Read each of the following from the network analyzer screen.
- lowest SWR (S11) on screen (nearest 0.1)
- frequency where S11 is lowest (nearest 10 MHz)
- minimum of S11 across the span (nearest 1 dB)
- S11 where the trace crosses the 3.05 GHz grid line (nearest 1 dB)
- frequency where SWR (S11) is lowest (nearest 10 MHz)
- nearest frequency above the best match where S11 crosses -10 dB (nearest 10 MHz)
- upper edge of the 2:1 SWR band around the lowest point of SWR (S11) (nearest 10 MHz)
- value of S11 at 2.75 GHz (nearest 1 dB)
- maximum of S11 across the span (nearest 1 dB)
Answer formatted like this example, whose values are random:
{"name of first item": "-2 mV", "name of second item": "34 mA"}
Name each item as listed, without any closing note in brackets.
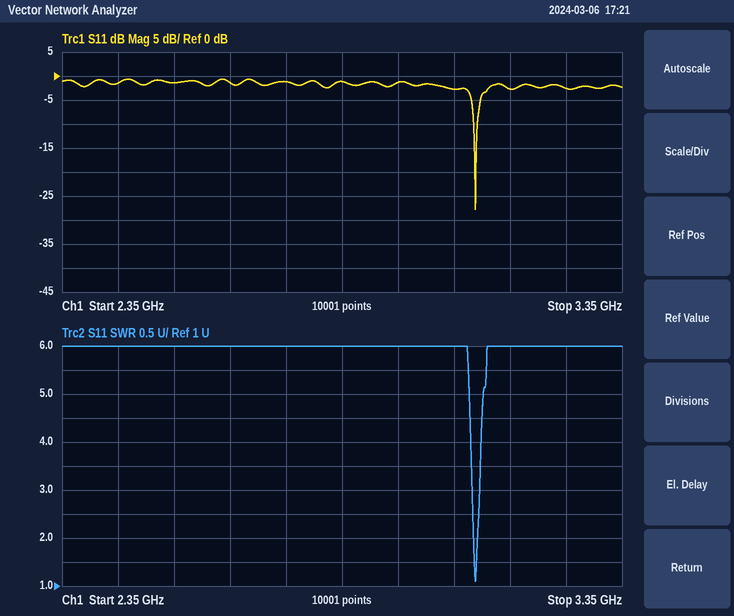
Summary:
{"lowest SWR (S11) on screen": "1.1", "frequency where S11 is lowest": "3.09 GHz", "minimum of S11 across the span": "-28 dB", "S11 where the trace crosses the 3.05 GHz grid line": "-3 dB", "frequency where SWR (S11) is lowest": "3.09 GHz", "nearest frequency above the best match where S11 crosses -10 dB": "3.09 GHz", "upper edge of the 2:1 SWR band around the lowest point of SWR (S11)": "3.09 GHz", "value of S11 at 2.75 GHz": "-1 dB", "maximum of S11 across the span": "-1 dB"}
